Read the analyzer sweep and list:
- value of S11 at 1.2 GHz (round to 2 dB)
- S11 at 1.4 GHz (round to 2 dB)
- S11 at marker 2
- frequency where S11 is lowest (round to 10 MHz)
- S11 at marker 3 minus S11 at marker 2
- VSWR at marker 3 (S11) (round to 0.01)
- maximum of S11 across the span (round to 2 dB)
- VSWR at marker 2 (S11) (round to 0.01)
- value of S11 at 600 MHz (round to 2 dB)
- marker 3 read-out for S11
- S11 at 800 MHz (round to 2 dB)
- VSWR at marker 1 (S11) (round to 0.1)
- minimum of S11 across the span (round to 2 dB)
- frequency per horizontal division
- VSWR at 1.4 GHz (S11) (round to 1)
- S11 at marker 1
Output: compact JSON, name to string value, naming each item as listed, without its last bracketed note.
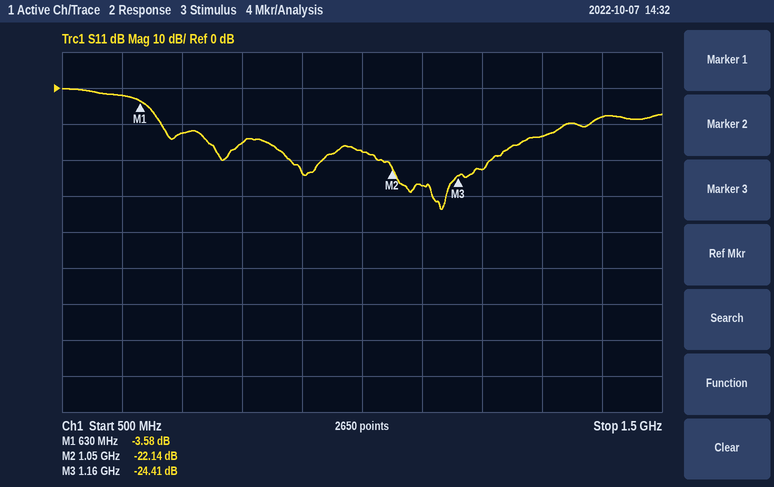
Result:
{"value of S11 at 1.2 GHz": "-22 dB", "S11 at 1.4 GHz": "-8 dB", "S11 at marker 2": "-22.14 dB", "frequency where S11 is lowest": "1.13 GHz", "S11 at marker 3 minus S11 at marker 2": "-2.27 dB", "VSWR at marker 3 (S11)": "1.13", "maximum of S11 across the span": "0 dB", "VSWR at marker 2 (S11)": "1.17", "value of S11 at 600 MHz": "-2 dB", "marker 3 read-out for S11": "-24.41 dB", "S11 at 800 MHz": "-16 dB", "VSWR at marker 1 (S11)": "4.9", "minimum of S11 across the span": "-34 dB", "frequency per horizontal division": "100 MHz", "VSWR at 1.4 GHz (S11)": "2", "S11 at marker 1": "-3.58 dB"}
